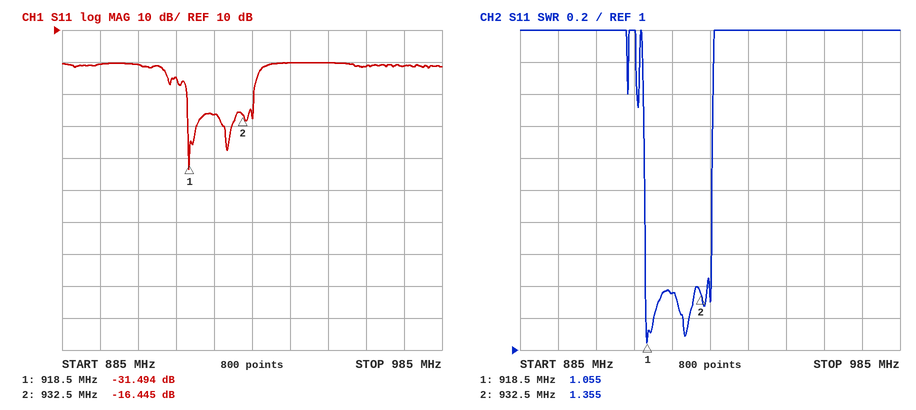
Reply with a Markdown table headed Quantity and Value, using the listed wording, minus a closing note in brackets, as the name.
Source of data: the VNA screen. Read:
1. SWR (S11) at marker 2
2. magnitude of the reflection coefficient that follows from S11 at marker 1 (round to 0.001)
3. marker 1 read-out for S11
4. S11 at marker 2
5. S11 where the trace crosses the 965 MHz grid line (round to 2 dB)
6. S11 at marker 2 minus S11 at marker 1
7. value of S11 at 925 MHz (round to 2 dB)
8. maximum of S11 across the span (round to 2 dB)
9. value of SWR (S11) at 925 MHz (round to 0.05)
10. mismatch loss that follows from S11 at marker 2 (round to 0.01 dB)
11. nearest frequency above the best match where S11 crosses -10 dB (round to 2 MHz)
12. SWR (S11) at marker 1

| Quantity | Value |
|---|---|
| SWR (S11) at marker 2 | 1.355 |
| magnitude of the reflection coefficient that follows from S11 at marker 1 | 0.027 |
| marker 1 read-out for S11 | -31.494 dB |
| S11 at marker 2 | -16.445 dB |
| S11 where the trace crosses the 965 MHz grid line | -2 dB |
| S11 at marker 2 minus S11 at marker 1 | 15.049 dB |
| value of S11 at 925 MHz | -16 dB |
| maximum of S11 across the span | 0 dB |
| value of SWR (S11) at 925 MHz | 1.35 |
| mismatch loss that follows from S11 at marker 2 | 0.10 dB |
| nearest frequency above the best match where S11 crosses -10 dB | 936 MHz |
| SWR (S11) at marker 1 | 1.055 |
